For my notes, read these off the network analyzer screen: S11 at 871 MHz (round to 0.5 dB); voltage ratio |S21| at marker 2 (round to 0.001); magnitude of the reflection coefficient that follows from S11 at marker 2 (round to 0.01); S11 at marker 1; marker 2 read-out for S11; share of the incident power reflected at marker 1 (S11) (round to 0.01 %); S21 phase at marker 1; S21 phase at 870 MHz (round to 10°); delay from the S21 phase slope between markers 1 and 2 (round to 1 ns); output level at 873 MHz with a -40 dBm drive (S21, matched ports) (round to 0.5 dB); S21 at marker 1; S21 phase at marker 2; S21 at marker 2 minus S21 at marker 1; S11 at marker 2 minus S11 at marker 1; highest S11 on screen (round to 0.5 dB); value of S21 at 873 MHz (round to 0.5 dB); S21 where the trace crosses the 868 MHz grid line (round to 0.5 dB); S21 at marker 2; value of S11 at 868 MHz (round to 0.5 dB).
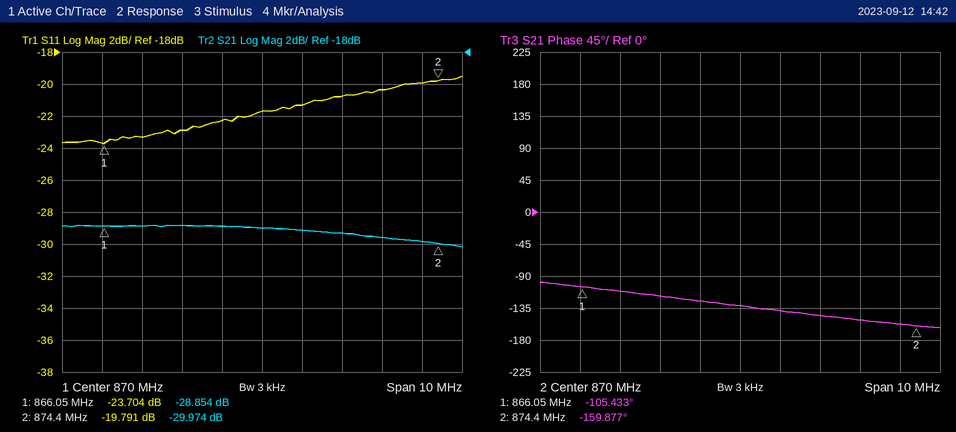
-21.5 dB
0.032
0.10
-23.704 dB
-19.791 dB
0.43 %
-105.433°
-130°
18 ns
-69.5 dBm
-28.854 dB
-159.877°
-1.120 dB
3.913 dB
-19.5 dB
-29.5 dB
-29.0 dB
-29.974 dB
-23.0 dB
